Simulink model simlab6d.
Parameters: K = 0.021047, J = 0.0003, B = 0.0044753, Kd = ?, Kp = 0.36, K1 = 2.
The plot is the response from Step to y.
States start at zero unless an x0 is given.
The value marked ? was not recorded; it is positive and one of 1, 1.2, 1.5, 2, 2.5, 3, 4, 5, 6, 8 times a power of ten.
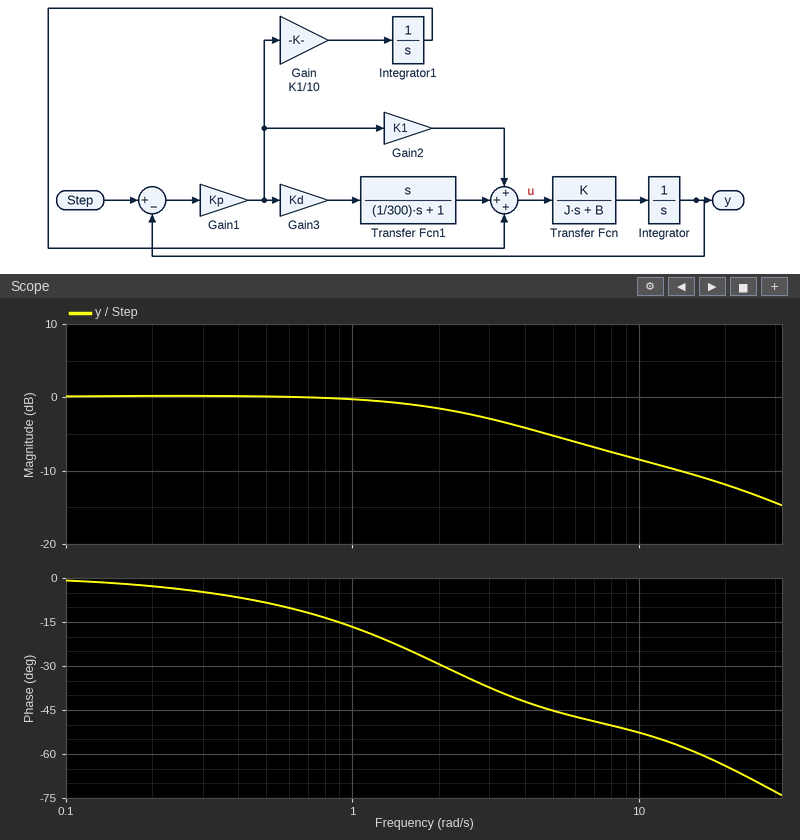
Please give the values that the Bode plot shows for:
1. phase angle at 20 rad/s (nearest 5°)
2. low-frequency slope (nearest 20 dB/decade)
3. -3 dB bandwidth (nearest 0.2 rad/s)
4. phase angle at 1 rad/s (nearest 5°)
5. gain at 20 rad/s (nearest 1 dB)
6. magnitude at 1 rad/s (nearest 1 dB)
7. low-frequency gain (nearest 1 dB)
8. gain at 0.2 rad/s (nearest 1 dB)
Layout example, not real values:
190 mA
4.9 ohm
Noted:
-65°
0 dB/decade
3.0 rad/s
-15°
-12 dB
0 dB
0 dB
0 dB
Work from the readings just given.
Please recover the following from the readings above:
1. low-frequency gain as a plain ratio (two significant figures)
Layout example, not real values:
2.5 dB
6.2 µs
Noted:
1.0
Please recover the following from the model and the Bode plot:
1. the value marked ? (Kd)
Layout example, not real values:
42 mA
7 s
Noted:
0.25
